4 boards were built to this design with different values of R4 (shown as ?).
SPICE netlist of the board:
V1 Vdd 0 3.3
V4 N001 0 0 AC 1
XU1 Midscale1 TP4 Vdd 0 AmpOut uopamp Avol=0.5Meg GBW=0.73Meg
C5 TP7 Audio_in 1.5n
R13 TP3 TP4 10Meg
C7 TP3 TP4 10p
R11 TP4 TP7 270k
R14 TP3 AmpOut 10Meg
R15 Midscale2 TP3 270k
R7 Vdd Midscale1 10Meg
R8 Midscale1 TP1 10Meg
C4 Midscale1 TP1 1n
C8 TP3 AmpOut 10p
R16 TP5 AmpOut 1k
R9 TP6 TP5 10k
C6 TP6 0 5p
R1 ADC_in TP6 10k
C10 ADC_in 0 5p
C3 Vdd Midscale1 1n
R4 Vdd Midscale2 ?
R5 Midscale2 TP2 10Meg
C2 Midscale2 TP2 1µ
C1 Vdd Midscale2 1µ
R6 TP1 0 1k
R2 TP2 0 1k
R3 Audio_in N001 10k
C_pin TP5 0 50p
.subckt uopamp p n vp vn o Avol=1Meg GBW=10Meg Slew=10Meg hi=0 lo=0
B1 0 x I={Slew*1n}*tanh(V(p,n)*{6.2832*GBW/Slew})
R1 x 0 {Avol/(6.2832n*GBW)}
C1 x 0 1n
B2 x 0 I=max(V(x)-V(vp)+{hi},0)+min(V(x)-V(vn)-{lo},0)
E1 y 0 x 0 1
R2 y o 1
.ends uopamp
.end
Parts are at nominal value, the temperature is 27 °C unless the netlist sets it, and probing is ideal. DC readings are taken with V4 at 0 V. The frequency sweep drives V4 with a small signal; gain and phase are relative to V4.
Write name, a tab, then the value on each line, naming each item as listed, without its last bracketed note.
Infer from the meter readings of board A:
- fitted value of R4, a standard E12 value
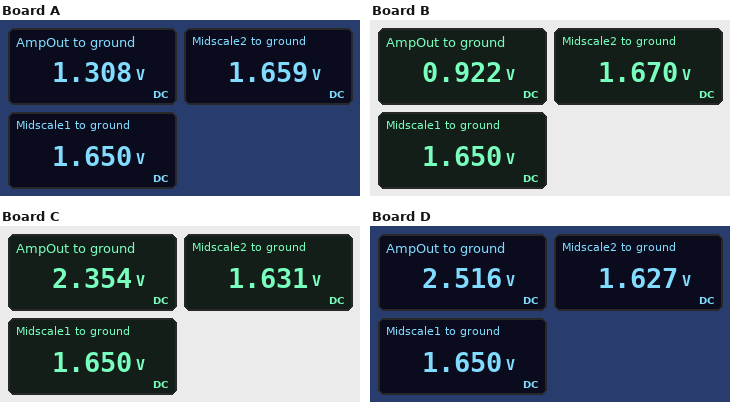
fitted value of R4, a standard E12 value	8.2 MΩ
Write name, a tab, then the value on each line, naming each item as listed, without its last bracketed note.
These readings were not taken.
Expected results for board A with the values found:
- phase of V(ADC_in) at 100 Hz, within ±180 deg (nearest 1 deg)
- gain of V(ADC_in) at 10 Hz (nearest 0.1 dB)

phase of V(ADC_in) at 100 Hz, within ±180 deg	-113 deg
gain of V(ADC_in) at 10 Hz	31.3 dB
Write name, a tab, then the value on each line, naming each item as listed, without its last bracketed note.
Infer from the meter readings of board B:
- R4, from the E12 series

R4, from the E12 series	6.8 MΩ
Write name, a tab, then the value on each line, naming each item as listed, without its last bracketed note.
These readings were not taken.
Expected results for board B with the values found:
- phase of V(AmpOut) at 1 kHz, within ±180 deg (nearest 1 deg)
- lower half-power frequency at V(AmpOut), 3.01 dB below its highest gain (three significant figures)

phase of V(AmpOut) at 1 kHz, within ±180 deg	110 deg
lower half-power frequency at V(AmpOut), 3.01 dB below its highest gain	187 Hz
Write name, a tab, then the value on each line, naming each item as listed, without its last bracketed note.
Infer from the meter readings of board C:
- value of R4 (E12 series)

value of R4	18 MΩ
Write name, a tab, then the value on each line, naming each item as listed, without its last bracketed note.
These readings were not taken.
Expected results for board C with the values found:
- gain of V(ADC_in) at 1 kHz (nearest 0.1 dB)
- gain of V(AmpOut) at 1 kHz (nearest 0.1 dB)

gain of V(ADC_in) at 1 kHz	52.9 dB
gain of V(AmpOut) at 1 kHz	52.9 dB
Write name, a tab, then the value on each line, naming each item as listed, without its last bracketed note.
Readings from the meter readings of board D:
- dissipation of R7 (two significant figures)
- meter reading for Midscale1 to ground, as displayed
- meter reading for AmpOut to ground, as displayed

dissipation of R7	270 nW
meter reading for Midscale1 to ground, as displayed	1.650 V
meter reading for AmpOut to ground, as displayed	2.516 V
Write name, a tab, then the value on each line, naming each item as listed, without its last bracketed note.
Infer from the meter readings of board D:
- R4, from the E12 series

R4, from the E12 series	22 MΩ
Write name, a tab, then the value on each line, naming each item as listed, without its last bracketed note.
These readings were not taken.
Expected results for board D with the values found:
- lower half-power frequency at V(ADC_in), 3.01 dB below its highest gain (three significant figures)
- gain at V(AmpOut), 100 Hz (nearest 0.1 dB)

lower half-power frequency at V(ADC_in), 3.01 dB below its highest gain	187 Hz
gain at V(AmpOut), 100 Hz	51.4 dB
